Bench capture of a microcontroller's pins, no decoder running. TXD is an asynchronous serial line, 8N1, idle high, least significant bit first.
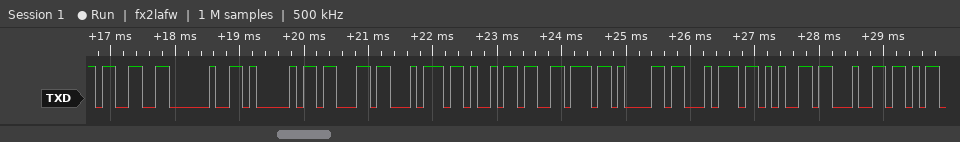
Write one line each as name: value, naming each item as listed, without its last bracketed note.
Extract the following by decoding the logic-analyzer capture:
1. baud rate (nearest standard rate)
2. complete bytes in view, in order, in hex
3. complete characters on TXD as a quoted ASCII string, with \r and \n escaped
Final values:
baud rate: 9600 baud
complete bytes in view, in order, in hex: 0x33 0x20 0x41 0x63 0x74 0x69 0x76 0x61 0x74 0x65 0x64
complete characters on TXD as a quoted ASCII string, with \r and \n escaped: "3 Activated"
